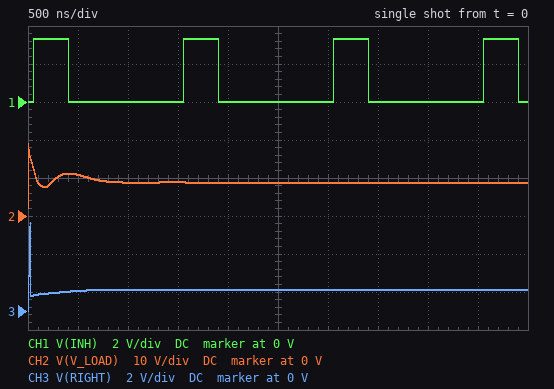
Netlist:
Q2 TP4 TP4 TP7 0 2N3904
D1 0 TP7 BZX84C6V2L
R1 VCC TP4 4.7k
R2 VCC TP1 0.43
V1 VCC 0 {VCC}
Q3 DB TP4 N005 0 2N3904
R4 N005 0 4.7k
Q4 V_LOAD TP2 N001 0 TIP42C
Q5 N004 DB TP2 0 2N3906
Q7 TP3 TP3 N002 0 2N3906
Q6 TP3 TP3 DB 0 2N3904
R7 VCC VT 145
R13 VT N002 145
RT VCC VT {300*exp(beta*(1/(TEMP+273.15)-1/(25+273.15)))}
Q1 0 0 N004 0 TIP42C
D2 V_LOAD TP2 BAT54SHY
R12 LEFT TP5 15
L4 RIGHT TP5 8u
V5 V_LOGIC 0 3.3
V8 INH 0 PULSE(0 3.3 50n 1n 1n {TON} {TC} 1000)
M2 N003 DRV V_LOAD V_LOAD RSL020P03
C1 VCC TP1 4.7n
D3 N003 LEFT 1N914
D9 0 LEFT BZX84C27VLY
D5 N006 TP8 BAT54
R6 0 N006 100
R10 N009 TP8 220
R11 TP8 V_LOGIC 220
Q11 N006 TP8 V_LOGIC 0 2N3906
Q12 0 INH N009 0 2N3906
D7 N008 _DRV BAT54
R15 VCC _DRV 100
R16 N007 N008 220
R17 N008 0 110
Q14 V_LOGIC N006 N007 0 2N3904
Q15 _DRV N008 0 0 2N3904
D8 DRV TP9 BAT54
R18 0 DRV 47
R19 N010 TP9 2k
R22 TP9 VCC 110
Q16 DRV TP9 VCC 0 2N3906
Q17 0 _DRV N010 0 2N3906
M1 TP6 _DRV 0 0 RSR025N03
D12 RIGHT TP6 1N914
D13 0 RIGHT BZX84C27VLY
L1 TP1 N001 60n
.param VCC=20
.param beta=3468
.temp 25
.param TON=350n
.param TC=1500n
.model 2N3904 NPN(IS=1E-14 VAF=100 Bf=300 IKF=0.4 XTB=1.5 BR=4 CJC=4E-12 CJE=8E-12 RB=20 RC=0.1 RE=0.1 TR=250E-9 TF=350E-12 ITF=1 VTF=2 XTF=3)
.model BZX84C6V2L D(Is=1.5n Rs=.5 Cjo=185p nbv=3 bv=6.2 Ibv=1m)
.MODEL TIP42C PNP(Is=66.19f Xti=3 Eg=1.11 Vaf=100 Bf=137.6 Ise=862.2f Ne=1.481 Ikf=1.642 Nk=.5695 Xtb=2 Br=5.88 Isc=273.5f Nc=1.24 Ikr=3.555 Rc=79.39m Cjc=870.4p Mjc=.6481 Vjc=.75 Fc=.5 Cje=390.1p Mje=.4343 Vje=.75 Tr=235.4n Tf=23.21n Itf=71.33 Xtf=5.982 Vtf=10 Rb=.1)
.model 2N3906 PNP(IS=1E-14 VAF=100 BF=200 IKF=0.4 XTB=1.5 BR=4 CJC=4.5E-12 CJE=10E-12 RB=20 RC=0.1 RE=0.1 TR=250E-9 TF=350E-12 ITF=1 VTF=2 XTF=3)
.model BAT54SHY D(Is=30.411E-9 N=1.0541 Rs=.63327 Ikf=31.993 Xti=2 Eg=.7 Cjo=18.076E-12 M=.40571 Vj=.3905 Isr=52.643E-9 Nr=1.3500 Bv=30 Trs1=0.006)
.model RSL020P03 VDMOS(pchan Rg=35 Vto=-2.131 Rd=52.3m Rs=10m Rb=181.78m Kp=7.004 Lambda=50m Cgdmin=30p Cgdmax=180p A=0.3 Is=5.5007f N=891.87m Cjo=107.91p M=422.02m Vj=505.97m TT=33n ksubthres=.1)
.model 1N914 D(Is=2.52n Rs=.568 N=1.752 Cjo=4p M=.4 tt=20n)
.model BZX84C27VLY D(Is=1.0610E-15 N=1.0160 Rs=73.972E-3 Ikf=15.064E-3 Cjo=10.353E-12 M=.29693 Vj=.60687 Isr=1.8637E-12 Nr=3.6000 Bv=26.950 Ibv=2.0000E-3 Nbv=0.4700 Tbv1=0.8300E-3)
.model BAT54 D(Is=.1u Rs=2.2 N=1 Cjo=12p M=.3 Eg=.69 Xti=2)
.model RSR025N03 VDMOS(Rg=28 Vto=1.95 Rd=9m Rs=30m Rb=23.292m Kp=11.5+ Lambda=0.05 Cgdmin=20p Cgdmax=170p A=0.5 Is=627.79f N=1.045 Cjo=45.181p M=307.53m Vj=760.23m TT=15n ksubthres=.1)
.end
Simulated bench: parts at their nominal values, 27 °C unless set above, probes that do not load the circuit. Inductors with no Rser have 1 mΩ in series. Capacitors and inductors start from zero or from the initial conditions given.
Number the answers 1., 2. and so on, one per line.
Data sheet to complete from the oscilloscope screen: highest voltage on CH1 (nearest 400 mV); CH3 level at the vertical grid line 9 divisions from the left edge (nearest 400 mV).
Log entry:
1. 3.2 V
2. 1.2 V
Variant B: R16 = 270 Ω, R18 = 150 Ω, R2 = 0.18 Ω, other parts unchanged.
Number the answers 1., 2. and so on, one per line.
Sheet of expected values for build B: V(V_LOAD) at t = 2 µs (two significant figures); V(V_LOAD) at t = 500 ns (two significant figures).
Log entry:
1. 14 V
2. 15 V
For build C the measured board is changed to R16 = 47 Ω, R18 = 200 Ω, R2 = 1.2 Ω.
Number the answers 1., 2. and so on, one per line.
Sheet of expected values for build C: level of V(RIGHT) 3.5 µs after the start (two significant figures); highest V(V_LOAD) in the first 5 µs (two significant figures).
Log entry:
1. 1.0 V
2. 20 V
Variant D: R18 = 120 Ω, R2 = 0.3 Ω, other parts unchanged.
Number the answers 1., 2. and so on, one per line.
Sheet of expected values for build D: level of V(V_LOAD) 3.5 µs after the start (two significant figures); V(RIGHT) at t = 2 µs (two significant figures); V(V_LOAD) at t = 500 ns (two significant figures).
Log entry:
1. 11 V
2. 1.2 V
3. 12 V
